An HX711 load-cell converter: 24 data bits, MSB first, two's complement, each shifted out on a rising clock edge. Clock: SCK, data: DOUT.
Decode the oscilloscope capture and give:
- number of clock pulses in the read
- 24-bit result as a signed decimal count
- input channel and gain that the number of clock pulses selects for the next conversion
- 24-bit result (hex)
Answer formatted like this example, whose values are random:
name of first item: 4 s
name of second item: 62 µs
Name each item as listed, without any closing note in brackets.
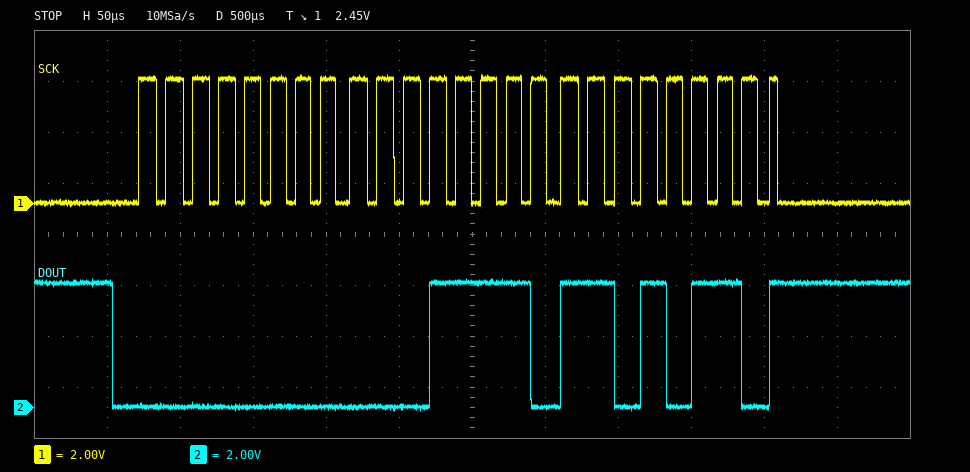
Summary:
number of clock pulses in the read: 25
24-bit result as a signed decimal count: 7894
input channel and gain that the number of clock pulses selects for the next conversion: channel A, gain 128
24-bit result: 0x001ED6
